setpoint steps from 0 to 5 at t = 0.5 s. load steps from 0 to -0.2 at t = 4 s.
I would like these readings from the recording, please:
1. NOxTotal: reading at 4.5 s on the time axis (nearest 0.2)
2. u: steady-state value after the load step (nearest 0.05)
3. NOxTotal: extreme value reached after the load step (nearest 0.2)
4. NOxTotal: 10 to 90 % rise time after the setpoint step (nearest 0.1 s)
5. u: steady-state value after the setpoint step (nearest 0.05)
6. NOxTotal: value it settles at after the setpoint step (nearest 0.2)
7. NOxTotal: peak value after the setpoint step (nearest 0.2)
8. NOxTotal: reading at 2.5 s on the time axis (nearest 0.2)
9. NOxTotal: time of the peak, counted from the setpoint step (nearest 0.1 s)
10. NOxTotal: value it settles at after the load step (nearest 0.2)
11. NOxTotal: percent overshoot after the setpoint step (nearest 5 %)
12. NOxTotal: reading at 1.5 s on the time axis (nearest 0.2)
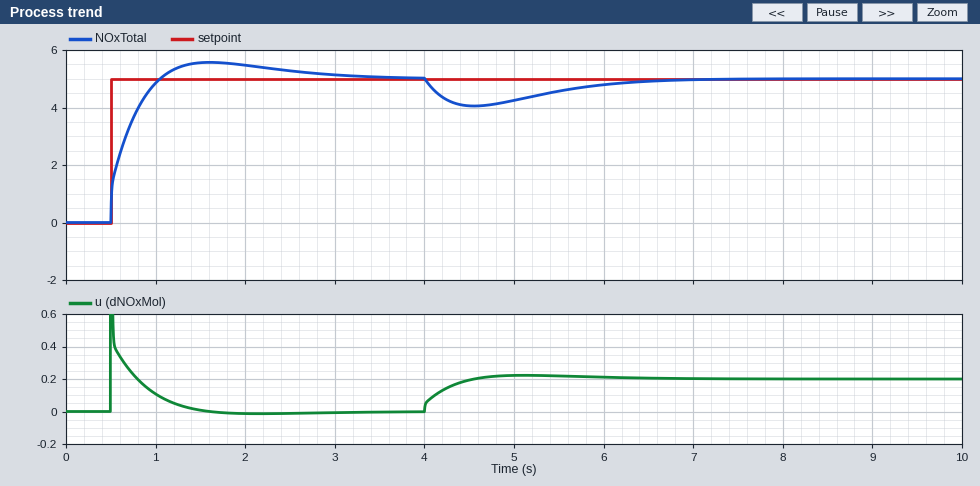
4.0
0.20
4.0
0.4 s
0.00
5.0
5.6
5.2
1.1 s
5.0
10 %
5.6
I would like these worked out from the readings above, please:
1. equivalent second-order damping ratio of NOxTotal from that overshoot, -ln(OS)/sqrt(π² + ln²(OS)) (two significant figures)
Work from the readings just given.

0.59
